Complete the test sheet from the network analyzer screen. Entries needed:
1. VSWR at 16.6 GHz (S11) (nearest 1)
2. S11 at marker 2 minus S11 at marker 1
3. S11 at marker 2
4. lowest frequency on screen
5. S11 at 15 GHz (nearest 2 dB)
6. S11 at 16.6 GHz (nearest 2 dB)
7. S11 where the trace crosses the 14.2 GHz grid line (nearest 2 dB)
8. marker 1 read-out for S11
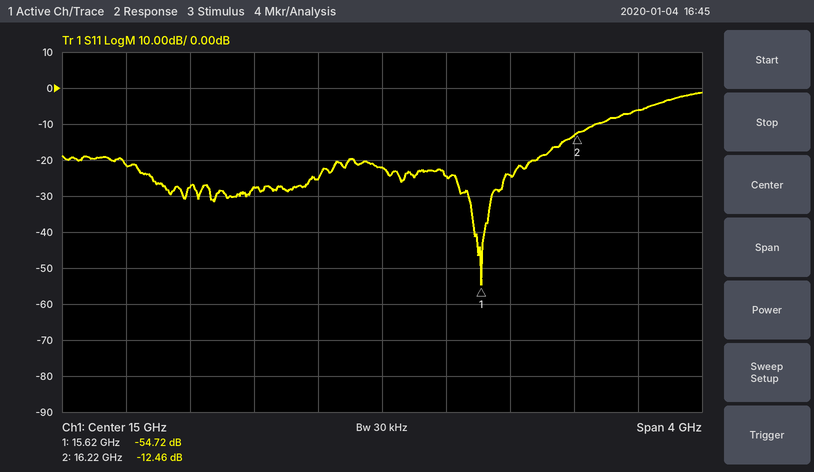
3
42.26 dB
-12.46 dB
13 GHz
-22 dB
-6 dB
-28 dB
-54.72 dB
